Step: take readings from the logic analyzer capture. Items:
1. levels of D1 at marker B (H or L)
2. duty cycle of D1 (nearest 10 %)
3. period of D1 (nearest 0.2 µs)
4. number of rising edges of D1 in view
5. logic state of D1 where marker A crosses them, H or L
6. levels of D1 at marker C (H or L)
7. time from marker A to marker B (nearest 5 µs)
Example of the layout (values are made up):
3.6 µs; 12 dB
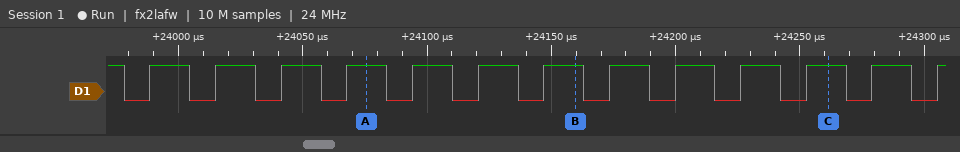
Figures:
D1=H; 60 %; 26.4 µs; 13; D1=H; D1=H; 85 µs
